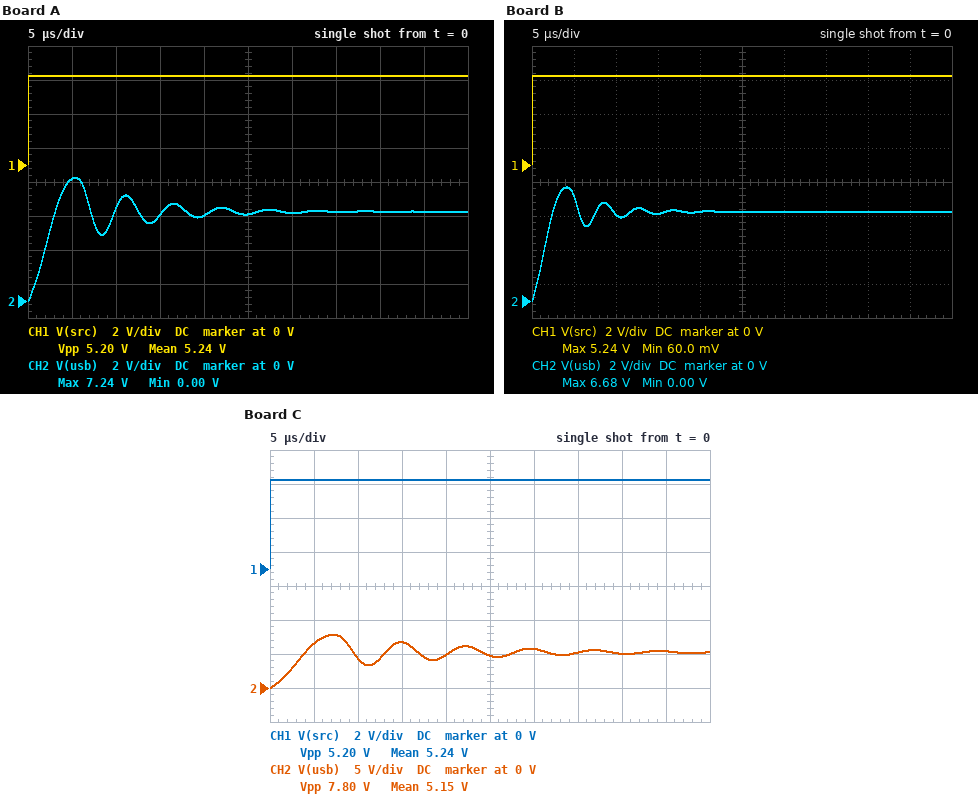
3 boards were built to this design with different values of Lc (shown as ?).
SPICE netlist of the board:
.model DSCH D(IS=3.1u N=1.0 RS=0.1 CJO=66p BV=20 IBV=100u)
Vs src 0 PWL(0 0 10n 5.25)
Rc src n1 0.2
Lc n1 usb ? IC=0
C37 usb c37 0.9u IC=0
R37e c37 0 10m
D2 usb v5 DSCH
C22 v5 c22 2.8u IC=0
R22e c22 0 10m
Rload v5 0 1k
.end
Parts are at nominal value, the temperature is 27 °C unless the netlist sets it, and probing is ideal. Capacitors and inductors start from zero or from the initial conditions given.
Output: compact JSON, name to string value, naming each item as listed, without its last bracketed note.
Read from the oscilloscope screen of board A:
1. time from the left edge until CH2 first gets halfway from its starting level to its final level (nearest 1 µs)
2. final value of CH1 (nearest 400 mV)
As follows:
{"time from the left edge until CH2 first gets halfway from its starting level to its final level": "2 µs", "final value of CH1": "5.2 V"}
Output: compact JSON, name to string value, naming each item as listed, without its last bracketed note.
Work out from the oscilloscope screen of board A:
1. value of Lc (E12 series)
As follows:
{"value of Lc": "820 nH"}
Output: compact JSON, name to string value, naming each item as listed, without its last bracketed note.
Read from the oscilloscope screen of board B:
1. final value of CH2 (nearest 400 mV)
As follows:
{"final value of CH2": "5.2 V"}
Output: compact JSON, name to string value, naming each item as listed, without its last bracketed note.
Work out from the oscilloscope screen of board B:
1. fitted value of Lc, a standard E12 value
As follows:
{"fitted value of Lc, a standard E12 value": "470 nH"}
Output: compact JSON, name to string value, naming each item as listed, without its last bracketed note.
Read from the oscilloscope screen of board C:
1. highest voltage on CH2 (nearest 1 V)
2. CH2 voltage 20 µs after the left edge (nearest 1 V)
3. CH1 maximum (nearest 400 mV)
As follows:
{"highest voltage on CH2": "8 V", "CH2 voltage 20 µs after the left edge": "5 V", "CH1 maximum": "5.2 V"}
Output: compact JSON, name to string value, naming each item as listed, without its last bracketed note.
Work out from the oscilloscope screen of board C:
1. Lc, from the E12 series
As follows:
{"Lc, from the E12 series": "1.5 µH"}
